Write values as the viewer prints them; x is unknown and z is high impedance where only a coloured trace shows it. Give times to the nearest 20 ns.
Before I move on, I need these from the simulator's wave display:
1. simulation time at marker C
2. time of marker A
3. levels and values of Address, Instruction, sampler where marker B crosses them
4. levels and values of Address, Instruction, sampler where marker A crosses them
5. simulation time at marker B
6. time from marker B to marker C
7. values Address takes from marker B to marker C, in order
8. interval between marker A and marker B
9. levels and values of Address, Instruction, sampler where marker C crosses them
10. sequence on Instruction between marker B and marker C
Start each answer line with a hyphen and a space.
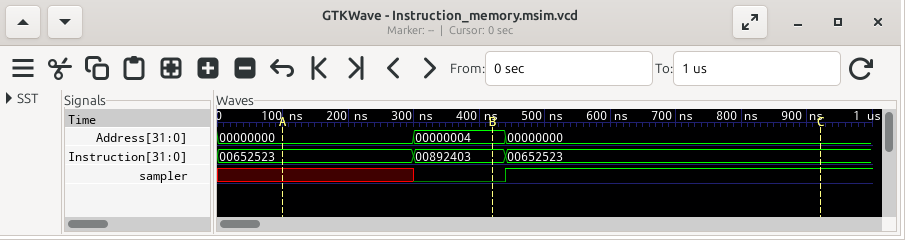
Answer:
- 920 ns
- 100 ns
- Address=00000004, Instruction=00892403, sampler=0
- Address=00000000, Instruction=00652523, sampler=x
- 420 ns
- 500 ns
- 00000004, 00000000
- 320 ns
- Address=00000000, Instruction=00652523, sampler=1
- 00892403, 00652523
